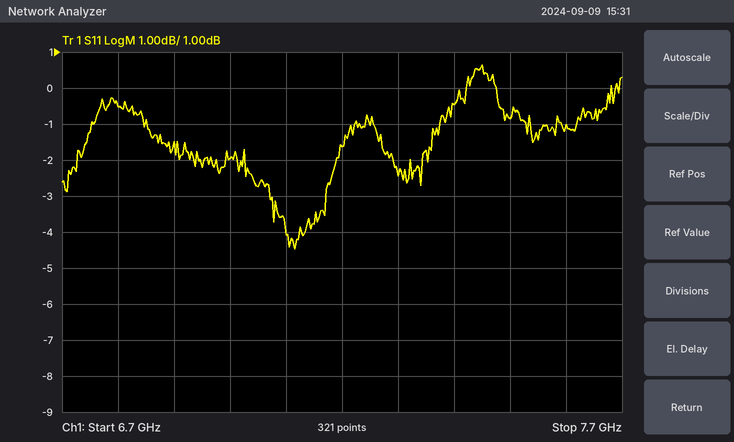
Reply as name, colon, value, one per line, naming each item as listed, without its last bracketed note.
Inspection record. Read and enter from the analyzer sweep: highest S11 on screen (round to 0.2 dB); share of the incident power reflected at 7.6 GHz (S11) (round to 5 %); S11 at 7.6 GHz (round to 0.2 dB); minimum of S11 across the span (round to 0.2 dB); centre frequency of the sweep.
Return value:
highest S11 on screen: 0.6 dB
share of the incident power reflected at 7.6 GHz (S11): 80 %
S11 at 7.6 GHz: -1.0 dB
minimum of S11 across the span: -4.4 dB
centre frequency of the sweep: 7.2 GHz
